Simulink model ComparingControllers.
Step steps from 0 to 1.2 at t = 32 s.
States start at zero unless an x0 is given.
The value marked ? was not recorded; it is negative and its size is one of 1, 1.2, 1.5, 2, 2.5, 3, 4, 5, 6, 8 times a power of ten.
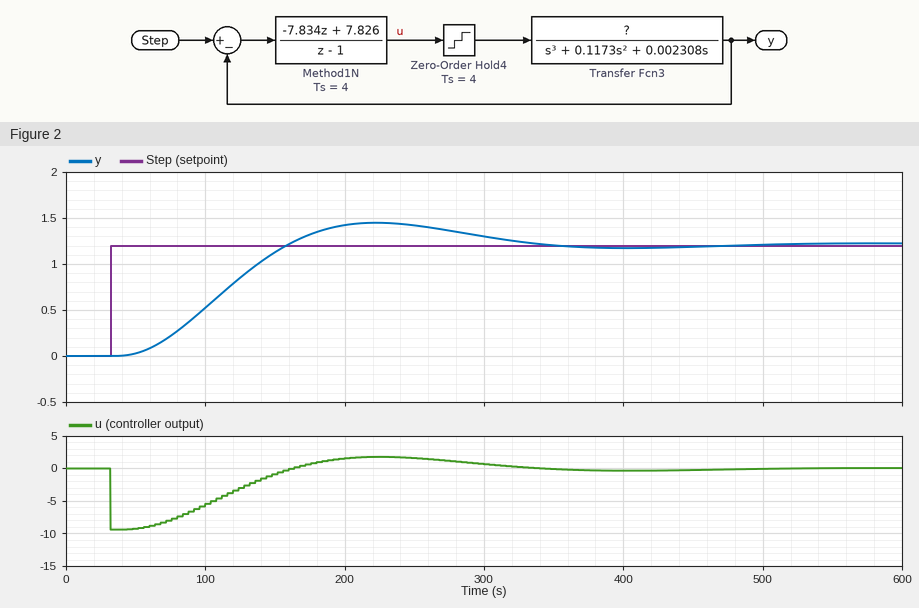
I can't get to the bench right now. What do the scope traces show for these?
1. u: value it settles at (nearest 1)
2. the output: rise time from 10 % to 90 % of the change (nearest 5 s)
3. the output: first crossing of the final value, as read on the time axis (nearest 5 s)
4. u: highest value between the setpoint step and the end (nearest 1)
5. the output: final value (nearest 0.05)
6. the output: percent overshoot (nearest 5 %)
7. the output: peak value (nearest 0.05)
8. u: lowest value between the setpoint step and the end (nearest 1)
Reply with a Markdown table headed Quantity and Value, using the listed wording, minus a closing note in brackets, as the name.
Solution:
| Quantity | Value |
|---|---|
| u: value it settles at | 0 |
| the output: rise time from 10 % to 90 % of the change | 80 s |
| the output: first crossing of the final value, as read on the time axis | 160 s |
| u: highest value between the setpoint step and the end | 2 |
| the output: final value | 1.20 |
| the output: percent overshoot | 20 % |
| the output: peak value | 1.45 |
| u: lowest value between the setpoint step and the end | -9 |
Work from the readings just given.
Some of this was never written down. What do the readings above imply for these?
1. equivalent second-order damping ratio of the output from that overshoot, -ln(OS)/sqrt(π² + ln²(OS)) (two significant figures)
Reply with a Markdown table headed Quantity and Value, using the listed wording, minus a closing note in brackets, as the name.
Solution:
| Quantity | Value |
|---|---|
| equivalent second-order damping ratio of the output from that overshoot, -ln(OS)/sqrt(π² + ln²(OS)) | 0.46 |
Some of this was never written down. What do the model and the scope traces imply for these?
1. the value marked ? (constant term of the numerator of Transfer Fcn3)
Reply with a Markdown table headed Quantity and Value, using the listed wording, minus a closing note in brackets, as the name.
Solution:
| Quantity | Value |
|---|---|
| the value marked ? | -5e-06 |
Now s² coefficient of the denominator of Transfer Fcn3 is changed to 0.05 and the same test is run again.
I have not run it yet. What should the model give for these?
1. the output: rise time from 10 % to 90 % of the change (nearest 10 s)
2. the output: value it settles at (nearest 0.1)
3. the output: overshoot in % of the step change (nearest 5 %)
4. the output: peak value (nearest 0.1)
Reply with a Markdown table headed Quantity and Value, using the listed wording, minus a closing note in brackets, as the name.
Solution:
| Quantity | Value |
|---|---|
| the output: rise time from 10 % to 90 % of the change | 60 s |
| the output: value it settles at | 1.2 |
| the output: overshoot in % of the step change | 10 % |
| the output: peak value | 1.3 |
